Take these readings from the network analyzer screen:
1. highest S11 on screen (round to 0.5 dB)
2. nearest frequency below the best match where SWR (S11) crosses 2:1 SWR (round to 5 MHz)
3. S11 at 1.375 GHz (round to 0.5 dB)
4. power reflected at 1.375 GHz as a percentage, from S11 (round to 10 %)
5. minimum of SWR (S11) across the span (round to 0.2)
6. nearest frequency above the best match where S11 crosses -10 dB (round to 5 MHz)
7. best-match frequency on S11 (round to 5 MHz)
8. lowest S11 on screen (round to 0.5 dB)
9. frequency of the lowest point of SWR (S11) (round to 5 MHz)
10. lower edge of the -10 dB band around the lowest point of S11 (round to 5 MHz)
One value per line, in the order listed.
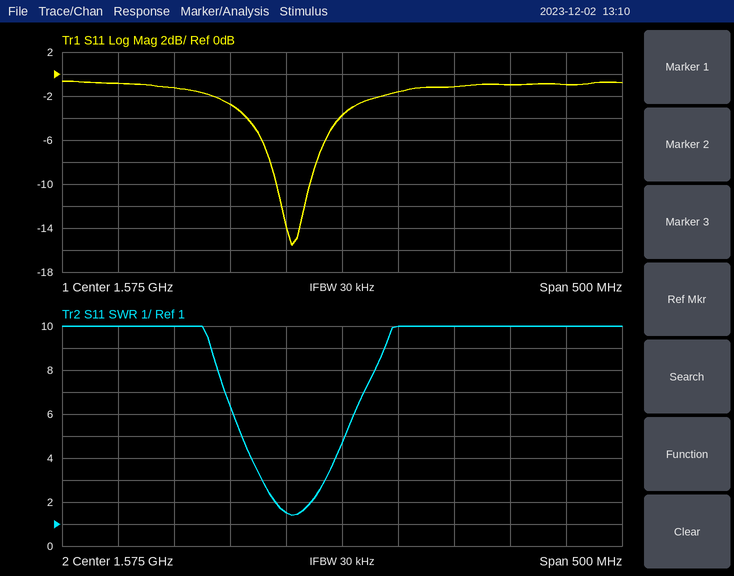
-0.5 dB
1.515 GHz
-1.0 dB
80 %
1.4
1.545 GHz
1.530 GHz
-15.5 dB
1.530 GHz
1.515 GHz
